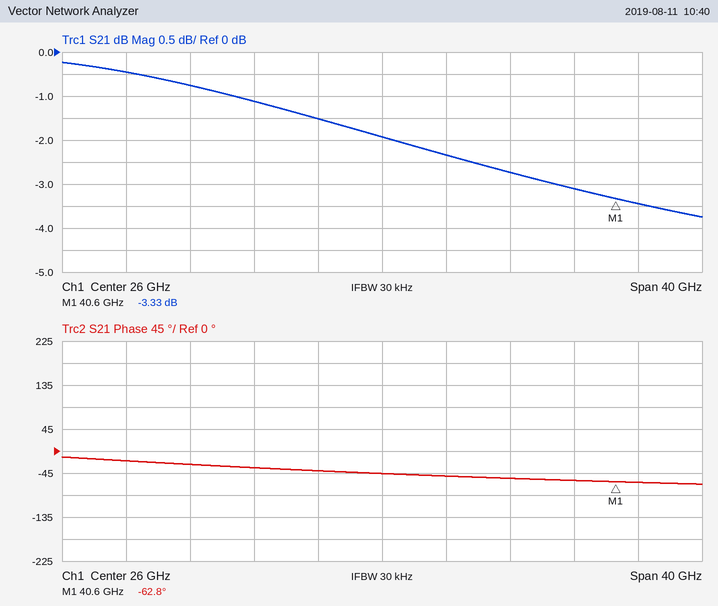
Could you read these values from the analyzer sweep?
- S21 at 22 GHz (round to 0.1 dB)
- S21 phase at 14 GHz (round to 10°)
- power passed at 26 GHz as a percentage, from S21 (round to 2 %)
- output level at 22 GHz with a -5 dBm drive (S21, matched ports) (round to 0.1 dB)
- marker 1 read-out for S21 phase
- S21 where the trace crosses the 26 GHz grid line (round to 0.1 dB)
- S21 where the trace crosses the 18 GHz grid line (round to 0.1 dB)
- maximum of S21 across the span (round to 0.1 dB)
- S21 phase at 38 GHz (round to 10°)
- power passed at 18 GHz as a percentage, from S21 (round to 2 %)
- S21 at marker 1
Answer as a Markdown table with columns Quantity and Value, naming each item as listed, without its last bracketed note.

| Quantity | Value |
|---|---|
| S21 at 22 GHz | -1.5 dB |
| S21 phase at 14 GHz | -30° |
| power passed at 26 GHz as a percentage, from S21 | 64 % |
| output level at 22 GHz with a -5 dBm drive (S21, matched ports) | -6.5 dBm |
| marker 1 read-out for S21 phase | -62.8° |
| S21 where the trace crosses the 26 GHz grid line | -1.9 dB |
| S21 where the trace crosses the 18 GHz grid line | -1.1 dB |
| maximum of S21 across the span | -0.2 dB |
| S21 phase at 38 GHz | -60° |
| power passed at 18 GHz as a percentage, from S21 | 78 % |
| S21 at marker 1 | -3.33 dB |
